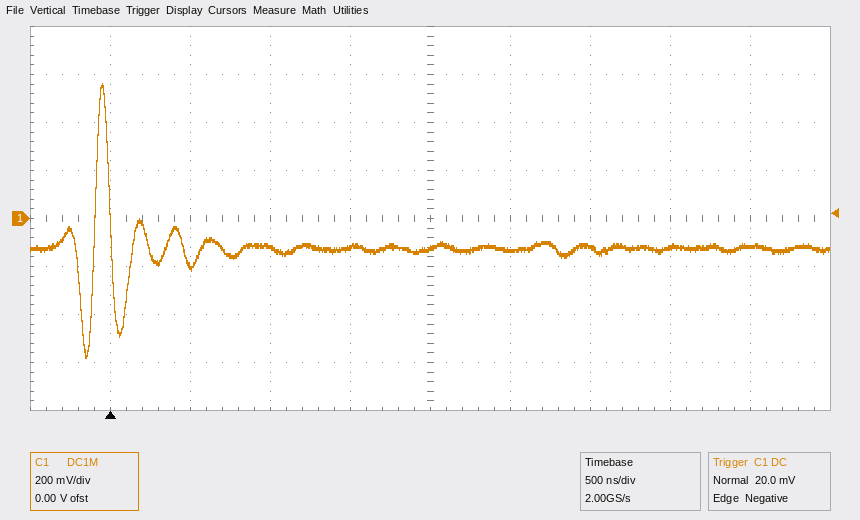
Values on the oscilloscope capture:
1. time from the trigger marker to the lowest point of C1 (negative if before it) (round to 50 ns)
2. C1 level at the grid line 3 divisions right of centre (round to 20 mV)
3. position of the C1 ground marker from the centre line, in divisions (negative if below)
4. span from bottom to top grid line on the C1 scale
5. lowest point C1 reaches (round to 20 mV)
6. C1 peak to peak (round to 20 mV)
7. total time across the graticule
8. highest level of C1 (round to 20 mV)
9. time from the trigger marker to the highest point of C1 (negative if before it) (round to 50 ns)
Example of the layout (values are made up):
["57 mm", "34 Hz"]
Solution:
["-150 ns", "-120 mV", "0.0 div", "1.6 V", "-580 mV", "1.14 V", "5 µs", "560 mV", "-50 ns"]
